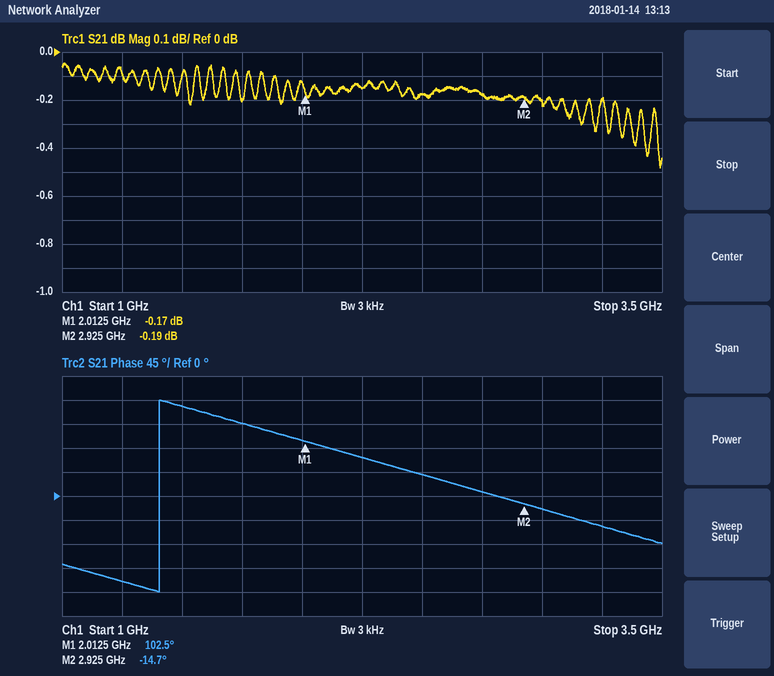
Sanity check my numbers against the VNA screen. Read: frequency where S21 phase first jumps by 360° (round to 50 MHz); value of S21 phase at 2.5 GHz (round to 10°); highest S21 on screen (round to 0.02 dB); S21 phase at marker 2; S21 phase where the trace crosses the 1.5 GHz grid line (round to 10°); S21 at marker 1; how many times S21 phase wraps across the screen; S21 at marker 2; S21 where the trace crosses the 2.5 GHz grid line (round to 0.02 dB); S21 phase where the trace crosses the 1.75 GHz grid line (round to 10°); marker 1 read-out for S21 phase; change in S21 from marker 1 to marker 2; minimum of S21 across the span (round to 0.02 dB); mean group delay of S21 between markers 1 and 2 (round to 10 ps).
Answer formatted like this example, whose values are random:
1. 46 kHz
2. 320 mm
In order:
1. 1.40 GHz
2. 40°
3. -0.04 dB
4. -14.7°
5. 170°
6. -0.17 dB
7. 1
8. -0.19 dB
9. -0.18 dB
10. 140°
11. 102.5°
12. -0.02 dB
13. -0.48 dB
14. 360 ps
